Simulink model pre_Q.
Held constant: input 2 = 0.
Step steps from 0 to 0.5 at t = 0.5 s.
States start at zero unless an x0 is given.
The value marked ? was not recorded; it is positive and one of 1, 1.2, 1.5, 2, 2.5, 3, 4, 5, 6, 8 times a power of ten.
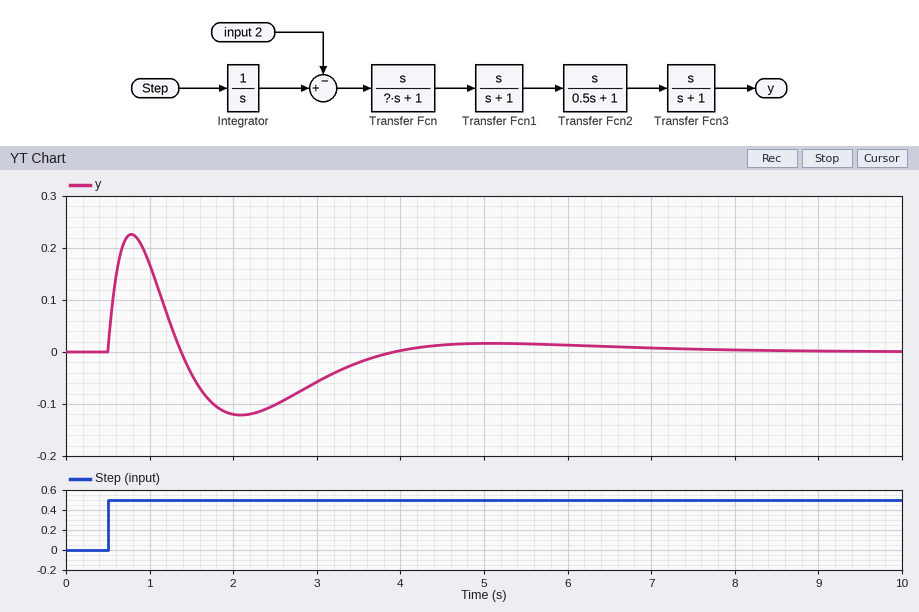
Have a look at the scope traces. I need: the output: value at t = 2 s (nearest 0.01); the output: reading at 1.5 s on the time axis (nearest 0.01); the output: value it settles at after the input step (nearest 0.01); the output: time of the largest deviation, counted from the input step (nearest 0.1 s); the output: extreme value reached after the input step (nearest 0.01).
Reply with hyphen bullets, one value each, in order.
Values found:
- -0.12
- -0.04
- 0.00
- 0.3 s
- 0.23
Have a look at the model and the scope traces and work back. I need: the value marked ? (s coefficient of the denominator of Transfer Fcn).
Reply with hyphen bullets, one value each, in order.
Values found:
- 0.5
